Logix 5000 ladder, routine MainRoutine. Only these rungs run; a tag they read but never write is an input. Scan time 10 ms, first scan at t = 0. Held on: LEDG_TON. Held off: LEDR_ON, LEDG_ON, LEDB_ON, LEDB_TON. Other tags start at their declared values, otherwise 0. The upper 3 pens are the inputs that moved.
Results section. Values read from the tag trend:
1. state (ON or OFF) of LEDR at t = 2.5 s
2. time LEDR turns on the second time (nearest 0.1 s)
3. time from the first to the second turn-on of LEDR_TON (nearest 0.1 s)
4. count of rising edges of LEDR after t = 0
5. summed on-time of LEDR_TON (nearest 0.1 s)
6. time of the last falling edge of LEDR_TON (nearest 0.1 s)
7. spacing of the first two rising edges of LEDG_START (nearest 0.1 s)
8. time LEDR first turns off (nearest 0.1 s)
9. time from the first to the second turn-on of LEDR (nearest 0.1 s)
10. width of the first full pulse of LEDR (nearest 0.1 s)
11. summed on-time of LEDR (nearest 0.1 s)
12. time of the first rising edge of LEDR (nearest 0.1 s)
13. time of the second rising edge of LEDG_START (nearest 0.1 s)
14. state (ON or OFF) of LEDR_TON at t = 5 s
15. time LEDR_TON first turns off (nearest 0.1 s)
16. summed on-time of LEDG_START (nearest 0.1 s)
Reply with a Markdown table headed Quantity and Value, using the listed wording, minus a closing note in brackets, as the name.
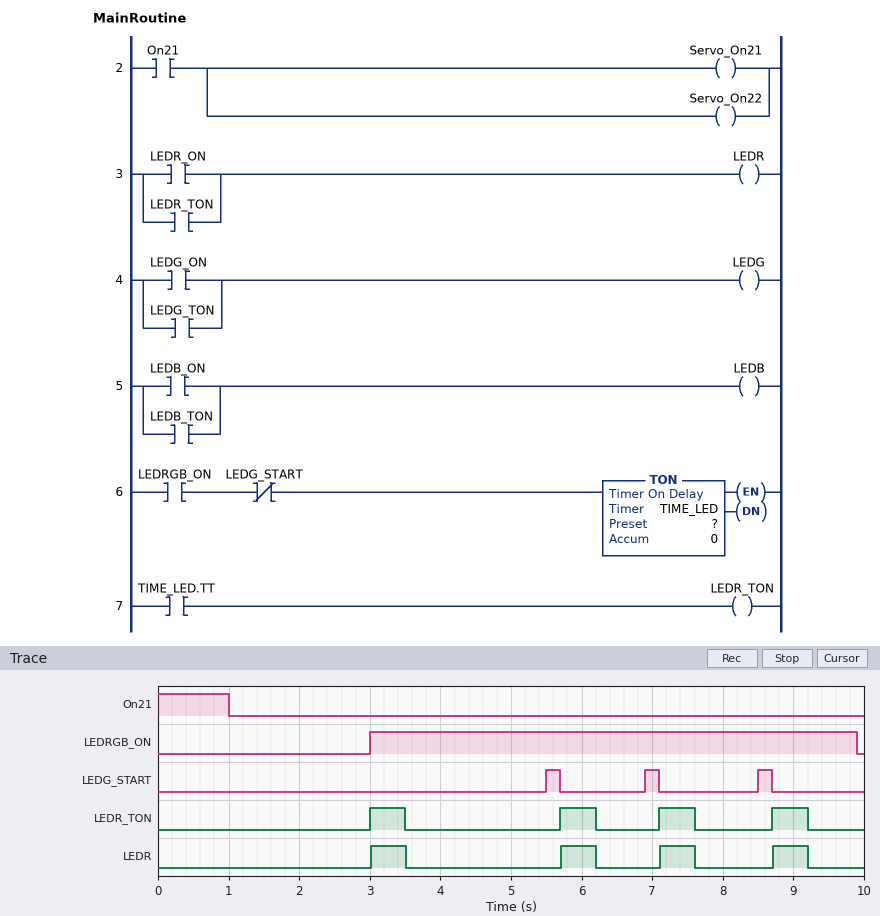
| Quantity | Value |
|---|---|
| state (ON or OFF) of LEDR at t = 2.5 s | OFF |
| time LEDR turns on the second time | 5.7 s |
| time from the first to the second turn-on of LEDR_TON | 2.7 s |
| count of rising edges of LEDR after t = 0 | 4 |
| summed on-time of LEDR_TON | 2.0 s |
| time of the last falling edge of LEDR_TON | 9.2 s |
| spacing of the first two rising edges of LEDG_START | 1.4 s |
| time LEDR first turns off | 3.5 s |
| time from the first to the second turn-on of LEDR | 2.7 s |
| width of the first full pulse of LEDR | 0.5 s |
| summed on-time of LEDR | 2.0 s |
| time of the first rising edge of LEDR | 3.0 s |
| time of the second rising edge of LEDG_START | 6.9 s |
| state (ON or OFF) of LEDR_TON at t = 5 s | OFF |
| time LEDR_TON first turns off | 3.5 s |
| summed on-time of LEDG_START | 0.6 s |
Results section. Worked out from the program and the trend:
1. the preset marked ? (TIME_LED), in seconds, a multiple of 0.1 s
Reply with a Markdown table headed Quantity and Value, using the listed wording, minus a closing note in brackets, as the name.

| Quantity | Value |
|---|---|
| the preset marked ? (TIME_LED), in seconds, a multiple of 0.1 s | 0.5 s |
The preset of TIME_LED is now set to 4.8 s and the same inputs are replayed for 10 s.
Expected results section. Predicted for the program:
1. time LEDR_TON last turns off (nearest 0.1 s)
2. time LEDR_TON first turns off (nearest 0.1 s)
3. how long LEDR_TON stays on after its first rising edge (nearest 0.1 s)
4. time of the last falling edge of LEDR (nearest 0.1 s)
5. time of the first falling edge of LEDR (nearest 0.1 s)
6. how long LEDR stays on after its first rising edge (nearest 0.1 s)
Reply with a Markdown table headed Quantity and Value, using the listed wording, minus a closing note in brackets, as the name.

| Quantity | Value |
|---|---|
| time LEDR_TON last turns off | 9.9 s |
| time LEDR_TON first turns off | 5.5 s |
| how long LEDR_TON stays on after its first rising edge | 2.5 s |
| time of the last falling edge of LEDR | 9.9 s |
| time of the first falling edge of LEDR | 5.5 s |
| how long LEDR stays on after its first rising edge | 2.5 s |
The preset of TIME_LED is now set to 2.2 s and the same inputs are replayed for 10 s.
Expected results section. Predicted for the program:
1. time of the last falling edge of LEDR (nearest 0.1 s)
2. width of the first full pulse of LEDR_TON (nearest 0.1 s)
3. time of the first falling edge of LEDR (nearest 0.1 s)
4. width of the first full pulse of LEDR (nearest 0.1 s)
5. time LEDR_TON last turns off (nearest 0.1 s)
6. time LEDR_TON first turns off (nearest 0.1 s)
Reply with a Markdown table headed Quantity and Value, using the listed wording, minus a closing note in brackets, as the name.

| Quantity | Value |
|---|---|
| time of the last falling edge of LEDR | 9.9 s |
| width of the first full pulse of LEDR_TON | 2.2 s |
| time of the first falling edge of LEDR | 5.2 s |
| width of the first full pulse of LEDR | 2.2 s |
| time LEDR_TON last turns off | 9.9 s |
| time LEDR_TON first turns off | 5.2 s |
